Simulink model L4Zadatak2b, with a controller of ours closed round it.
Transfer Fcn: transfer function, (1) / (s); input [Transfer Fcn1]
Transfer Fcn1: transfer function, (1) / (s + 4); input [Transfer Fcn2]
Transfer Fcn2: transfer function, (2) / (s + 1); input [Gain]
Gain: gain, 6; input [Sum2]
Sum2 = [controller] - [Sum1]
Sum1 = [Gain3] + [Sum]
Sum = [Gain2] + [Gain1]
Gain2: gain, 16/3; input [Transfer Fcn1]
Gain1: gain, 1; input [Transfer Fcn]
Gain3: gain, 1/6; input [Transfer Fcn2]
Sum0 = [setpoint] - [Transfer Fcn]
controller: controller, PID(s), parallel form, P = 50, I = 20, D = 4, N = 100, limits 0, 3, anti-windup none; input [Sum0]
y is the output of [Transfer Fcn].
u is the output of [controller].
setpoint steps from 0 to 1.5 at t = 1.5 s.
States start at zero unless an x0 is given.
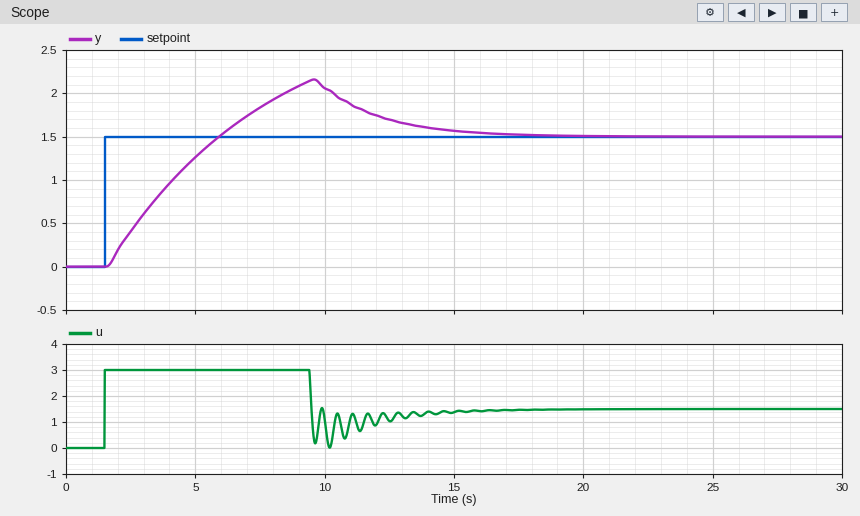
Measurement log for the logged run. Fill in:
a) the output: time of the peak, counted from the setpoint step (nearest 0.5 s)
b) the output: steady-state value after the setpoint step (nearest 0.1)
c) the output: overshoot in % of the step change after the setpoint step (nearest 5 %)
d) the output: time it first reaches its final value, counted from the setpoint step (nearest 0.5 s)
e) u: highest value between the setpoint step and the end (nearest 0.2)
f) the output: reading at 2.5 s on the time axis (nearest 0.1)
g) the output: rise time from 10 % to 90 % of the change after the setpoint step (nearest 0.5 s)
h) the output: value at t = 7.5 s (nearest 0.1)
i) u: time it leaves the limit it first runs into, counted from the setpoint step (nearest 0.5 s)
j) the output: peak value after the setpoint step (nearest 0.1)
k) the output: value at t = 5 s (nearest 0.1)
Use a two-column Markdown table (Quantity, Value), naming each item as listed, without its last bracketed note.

| Quantity | Value |
|---|---|
| the output: time of the peak, counted from the setpoint step | 8.0 s |
| the output: steady-state value after the setpoint step | 1.5 |
| the output: overshoot in % of the step change after the setpoint step | 45 % |
| the output: time it first reaches its final value, counted from the setpoint step | 4.5 s |
| u: highest value between the setpoint step and the end | 3.0 |
| the output: reading at 2.5 s on the time axis | 0.4 |
| the output: rise time from 10 % to 90 % of the change after the setpoint step | 3.5 s |
| the output: value at t = 7.5 s | 1.8 |
| u: time it leaves the limit it first runs into, counted from the setpoint step | 8.0 s |
| the output: peak value after the setpoint step | 2.2 |
| the output: value at t = 5 s | 1.3 |
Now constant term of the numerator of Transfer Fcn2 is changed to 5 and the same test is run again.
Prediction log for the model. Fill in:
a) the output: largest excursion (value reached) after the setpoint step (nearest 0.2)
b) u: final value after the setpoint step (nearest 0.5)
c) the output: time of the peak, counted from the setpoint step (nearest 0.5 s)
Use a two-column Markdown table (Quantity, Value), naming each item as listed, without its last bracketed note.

| Quantity | Value |
|---|---|
| the output: largest excursion (value reached) after the setpoint step | 2.2 |
| u: final value after the setpoint step | 1.5 |
| the output: time of the peak, counted from the setpoint step | 7.5 s |
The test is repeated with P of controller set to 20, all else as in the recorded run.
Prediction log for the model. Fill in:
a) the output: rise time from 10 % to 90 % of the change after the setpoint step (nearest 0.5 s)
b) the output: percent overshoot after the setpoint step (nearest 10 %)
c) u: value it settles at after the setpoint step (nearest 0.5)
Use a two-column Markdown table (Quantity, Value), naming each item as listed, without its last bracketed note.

| Quantity | Value |
|---|---|
| the output: rise time from 10 % to 90 % of the change after the setpoint step | 3.5 s |
| the output: percent overshoot after the setpoint step | 50 % |
| u: value it settles at after the setpoint step | 1.5 |
